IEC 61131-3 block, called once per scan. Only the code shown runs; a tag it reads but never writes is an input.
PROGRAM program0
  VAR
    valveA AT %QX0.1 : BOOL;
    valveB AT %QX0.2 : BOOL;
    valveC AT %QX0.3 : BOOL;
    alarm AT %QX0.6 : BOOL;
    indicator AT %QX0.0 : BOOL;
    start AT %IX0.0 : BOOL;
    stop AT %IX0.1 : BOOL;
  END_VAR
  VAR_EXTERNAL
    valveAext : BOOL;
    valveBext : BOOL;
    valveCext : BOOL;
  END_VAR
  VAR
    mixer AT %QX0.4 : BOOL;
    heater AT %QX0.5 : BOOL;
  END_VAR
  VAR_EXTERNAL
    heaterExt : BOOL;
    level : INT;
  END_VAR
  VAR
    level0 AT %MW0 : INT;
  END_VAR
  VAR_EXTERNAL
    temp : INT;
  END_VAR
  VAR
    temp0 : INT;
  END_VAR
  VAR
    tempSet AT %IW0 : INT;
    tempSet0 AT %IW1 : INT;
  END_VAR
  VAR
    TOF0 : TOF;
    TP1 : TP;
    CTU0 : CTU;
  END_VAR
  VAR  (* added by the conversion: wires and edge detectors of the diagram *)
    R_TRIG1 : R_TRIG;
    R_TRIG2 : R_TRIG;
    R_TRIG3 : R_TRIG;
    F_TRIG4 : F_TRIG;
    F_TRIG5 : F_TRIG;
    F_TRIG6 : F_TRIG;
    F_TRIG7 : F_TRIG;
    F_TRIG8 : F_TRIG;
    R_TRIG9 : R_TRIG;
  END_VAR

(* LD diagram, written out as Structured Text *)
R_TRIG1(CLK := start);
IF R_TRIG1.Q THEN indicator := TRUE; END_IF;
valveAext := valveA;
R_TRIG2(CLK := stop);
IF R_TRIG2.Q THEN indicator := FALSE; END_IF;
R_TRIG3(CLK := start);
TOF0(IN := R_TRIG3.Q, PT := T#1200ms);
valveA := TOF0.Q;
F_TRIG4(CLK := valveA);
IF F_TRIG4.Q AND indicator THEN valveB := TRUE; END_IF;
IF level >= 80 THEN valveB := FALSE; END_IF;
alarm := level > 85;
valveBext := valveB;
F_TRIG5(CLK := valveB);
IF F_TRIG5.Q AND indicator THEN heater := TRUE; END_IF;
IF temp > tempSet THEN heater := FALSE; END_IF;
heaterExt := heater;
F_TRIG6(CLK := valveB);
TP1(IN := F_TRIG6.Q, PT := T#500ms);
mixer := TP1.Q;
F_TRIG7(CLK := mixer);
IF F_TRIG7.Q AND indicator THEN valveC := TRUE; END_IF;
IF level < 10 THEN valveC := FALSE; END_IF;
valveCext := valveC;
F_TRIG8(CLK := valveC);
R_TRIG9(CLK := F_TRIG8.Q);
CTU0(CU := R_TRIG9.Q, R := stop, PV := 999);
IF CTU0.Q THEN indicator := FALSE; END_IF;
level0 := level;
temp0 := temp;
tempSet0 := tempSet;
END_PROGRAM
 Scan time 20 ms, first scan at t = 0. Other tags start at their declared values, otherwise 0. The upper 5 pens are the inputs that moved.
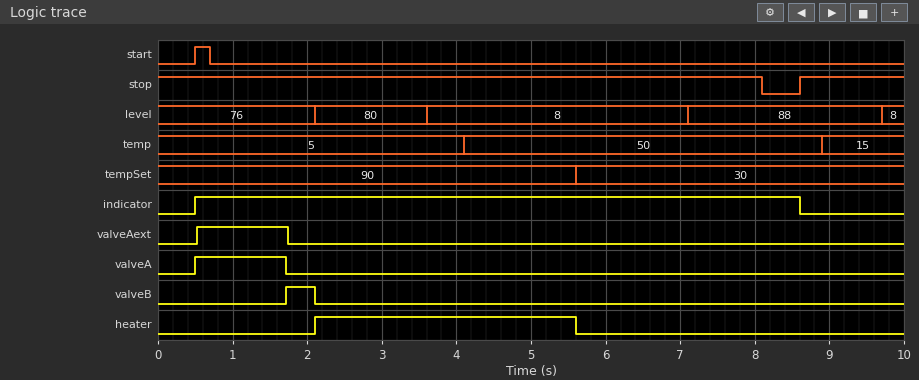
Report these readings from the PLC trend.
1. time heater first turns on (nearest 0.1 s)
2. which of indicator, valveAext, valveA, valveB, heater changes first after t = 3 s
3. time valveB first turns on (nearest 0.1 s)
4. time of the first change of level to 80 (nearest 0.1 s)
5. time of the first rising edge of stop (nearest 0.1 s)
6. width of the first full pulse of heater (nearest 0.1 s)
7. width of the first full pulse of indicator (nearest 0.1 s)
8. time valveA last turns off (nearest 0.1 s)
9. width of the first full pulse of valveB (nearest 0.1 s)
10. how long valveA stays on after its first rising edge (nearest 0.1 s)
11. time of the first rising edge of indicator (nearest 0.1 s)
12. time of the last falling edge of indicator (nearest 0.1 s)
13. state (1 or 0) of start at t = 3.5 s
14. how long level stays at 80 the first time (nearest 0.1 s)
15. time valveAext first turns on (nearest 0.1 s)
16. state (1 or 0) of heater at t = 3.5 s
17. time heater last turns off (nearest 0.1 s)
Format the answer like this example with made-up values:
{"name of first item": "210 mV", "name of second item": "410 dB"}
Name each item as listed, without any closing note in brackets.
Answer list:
{"time heater first turns on": "2.1 s", "which of indicator, valveAext, valveA, valveB, heater changes first after t = 3 s": "heater", "time valveB first turns on": "1.7 s", "time of the first change of level to 80": "2.1 s", "time of the first rising edge of stop": "8.6 s", "width of the first full pulse of heater": "3.5 s", "width of the first full pulse of indicator": "8.1 s", "time valveA last turns off": "1.7 s", "width of the first full pulse of valveB": "0.4 s", "how long valveA stays on after its first rising edge": "1.2 s", "time of the first rising edge of indicator": "0.5 s", "time of the last falling edge of indicator": "8.6 s", "state (1 or 0) of start at t = 3.5 s": "0", "how long level stays at 80 the first time": "1.5 s", "time valveAext first turns on": "0.5 s", "state (1 or 0) of heater at t = 3.5 s": "1", "time heater last turns off": "5.6 s"}
